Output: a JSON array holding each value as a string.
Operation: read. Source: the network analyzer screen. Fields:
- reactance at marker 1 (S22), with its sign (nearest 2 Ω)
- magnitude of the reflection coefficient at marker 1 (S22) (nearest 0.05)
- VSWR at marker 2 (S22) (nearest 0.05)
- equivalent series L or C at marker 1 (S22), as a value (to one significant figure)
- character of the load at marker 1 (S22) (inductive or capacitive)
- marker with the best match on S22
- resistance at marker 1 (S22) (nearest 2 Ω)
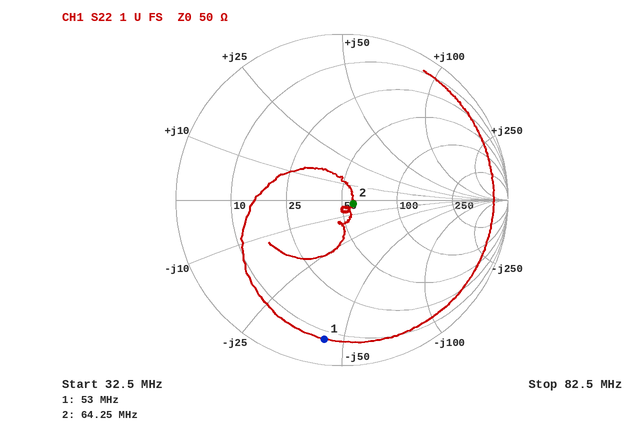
["-44 Ω", "0.85", "1.15", "70 pF", "capacitive", "marker 2", "8 Ω"]
